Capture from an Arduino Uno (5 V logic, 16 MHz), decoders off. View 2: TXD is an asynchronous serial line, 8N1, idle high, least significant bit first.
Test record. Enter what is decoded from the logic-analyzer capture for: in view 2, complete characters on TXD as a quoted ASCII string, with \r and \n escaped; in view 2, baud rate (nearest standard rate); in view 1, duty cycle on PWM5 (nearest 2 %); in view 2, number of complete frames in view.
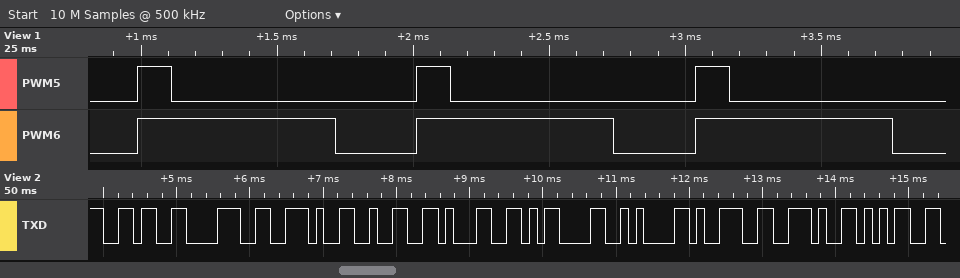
"68.21\r\n9.5"
9600 baud
12 %
10
